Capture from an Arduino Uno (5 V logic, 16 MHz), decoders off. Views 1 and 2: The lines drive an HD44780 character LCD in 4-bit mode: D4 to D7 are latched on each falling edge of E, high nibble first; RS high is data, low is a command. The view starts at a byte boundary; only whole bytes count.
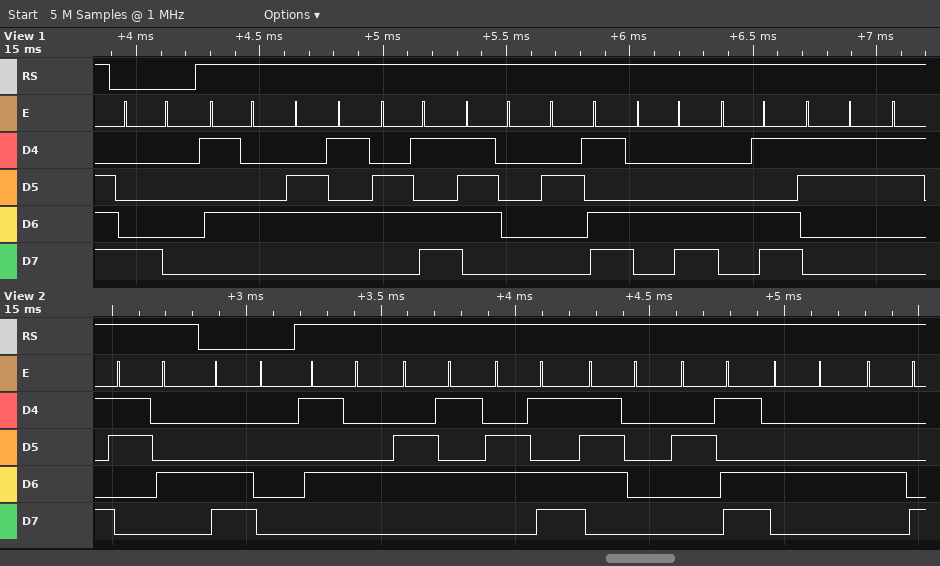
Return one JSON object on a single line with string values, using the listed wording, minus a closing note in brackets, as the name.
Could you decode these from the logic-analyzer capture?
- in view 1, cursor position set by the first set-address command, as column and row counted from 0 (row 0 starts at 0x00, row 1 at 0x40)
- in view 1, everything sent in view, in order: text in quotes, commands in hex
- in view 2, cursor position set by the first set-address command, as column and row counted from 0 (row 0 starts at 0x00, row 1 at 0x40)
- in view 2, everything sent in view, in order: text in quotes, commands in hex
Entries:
{"in view 1, cursor position set by the first set-address command, as column and row counted from 0": "column 0, row 0", "in view 1, everything sent in view, in order: text in quotes, commands in hex": "0x80 \"Temp-LM3\"", "in view 2, cursor position set by the first set-address command, as column and row counted from 0": "column 0, row 1", "in view 2, everything sent in view, in order: text in quotes, commands in hex": "\"4\" 0xC0 \"Temp-DH\""}
